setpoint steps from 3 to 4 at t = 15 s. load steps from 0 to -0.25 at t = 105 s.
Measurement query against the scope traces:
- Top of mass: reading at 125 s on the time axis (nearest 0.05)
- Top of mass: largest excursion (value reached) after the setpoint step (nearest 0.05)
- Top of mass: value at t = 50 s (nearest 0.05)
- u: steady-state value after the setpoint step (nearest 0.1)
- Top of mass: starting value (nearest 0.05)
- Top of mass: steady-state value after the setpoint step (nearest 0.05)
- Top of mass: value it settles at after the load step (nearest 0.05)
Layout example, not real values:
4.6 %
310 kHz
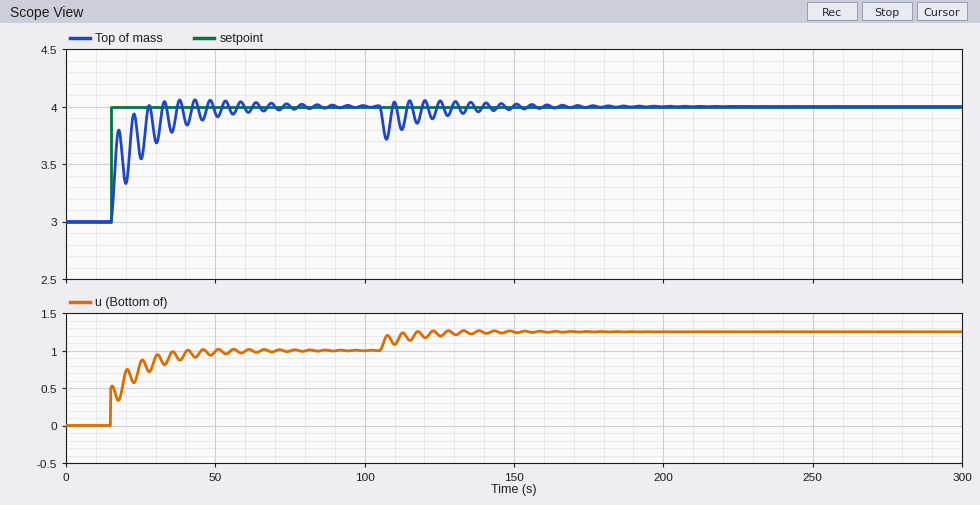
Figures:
4.05
4.05
3.95
1.0
3.00
4.00
4.00
